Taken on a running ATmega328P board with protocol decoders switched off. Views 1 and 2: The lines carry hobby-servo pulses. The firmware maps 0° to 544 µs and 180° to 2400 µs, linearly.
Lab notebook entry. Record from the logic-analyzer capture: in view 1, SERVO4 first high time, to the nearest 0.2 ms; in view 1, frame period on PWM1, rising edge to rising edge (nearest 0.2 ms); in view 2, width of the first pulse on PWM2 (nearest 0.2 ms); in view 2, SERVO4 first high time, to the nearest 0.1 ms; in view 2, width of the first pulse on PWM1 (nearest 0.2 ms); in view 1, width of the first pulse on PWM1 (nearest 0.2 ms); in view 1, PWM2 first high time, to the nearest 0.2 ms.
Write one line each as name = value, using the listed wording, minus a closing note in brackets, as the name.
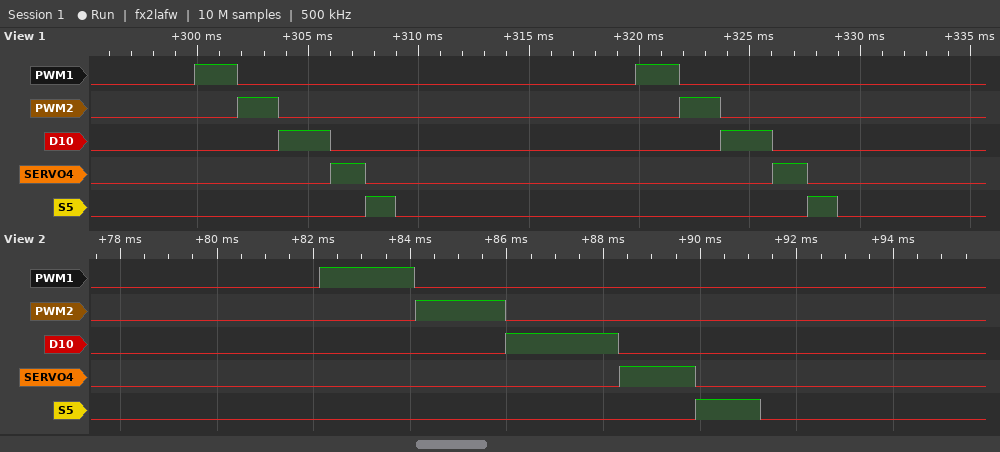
in view 1, SERVO4 first high time, to the nearest 0.2 ms = 1.6 ms
in view 1, frame period on PWM1, rising edge to rising edge = 20.0 ms
in view 2, width of the first pulse on PWM2 = 1.8 ms
in view 2, SERVO4 first high time, to the nearest 0.1 ms = 1.6 ms
in view 2, width of the first pulse on PWM1 = 2.0 ms
in view 1, width of the first pulse on PWM1 = 2.0 ms
in view 1, PWM2 first high time, to the nearest 0.2 ms = 1.8 ms
